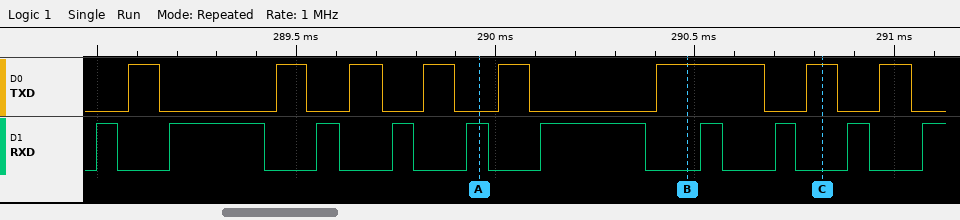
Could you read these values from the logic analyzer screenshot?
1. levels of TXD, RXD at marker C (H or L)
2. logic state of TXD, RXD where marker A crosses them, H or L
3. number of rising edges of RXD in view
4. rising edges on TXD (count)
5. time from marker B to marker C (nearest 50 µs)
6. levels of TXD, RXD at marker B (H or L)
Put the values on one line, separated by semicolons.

TXD=H, RXD=L; TXD=L, RXD=H; 10; 8; 350 µs; TXD=H, RXD=L
